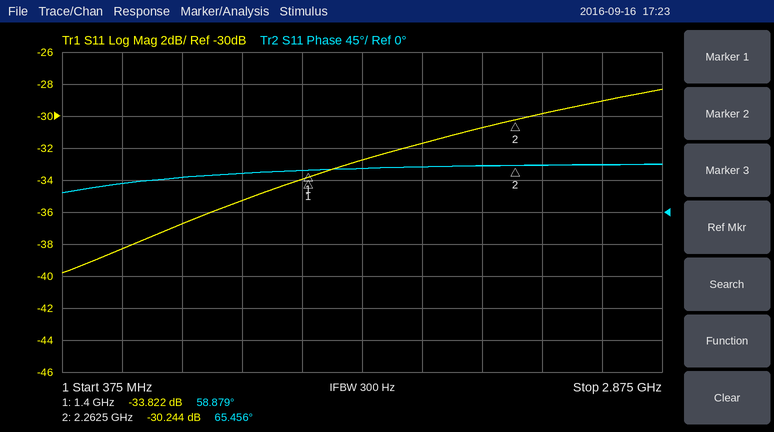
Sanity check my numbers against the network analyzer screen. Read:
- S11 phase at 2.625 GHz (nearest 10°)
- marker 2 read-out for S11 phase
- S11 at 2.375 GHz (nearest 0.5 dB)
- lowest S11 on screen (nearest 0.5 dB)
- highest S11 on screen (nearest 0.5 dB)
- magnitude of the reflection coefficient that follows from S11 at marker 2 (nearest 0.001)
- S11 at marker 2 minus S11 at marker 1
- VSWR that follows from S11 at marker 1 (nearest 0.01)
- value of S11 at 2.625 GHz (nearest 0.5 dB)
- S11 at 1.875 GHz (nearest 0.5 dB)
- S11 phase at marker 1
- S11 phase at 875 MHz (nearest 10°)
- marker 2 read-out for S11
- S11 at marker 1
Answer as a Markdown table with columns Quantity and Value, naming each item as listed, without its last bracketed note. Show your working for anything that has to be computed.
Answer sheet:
| Quantity | Value |
|---|---|
| S11 phase at 2.625 GHz | 70° |
| marker 2 read-out for S11 phase | 65.456° |
| S11 at 2.375 GHz | -30.0 dB |
| lowest S11 on screen | -40.0 dB |
| highest S11 on screen | -28.5 dB |
| magnitude of the reflection coefficient that follows from S11 at marker 2 | 10^(-30.244/20) ≈ 0.031 |
| S11 at marker 2 minus S11 at marker 1 | -30.244 − (-33.822) = 3.578 dB |
| VSWR that follows from S11 at marker 1 | (1 + 0.0204)/(1 − 0.0204) ≈ 1.04 |
| value of S11 at 2.625 GHz | -29.0 dB |
| S11 at 1.875 GHz | -31.5 dB |
| S11 phase at marker 1 | 58.879° |
| S11 phase at 875 MHz | 50° |
| marker 2 read-out for S11 | -30.244 dB |
| S11 at marker 1 | -33.822 dB |
